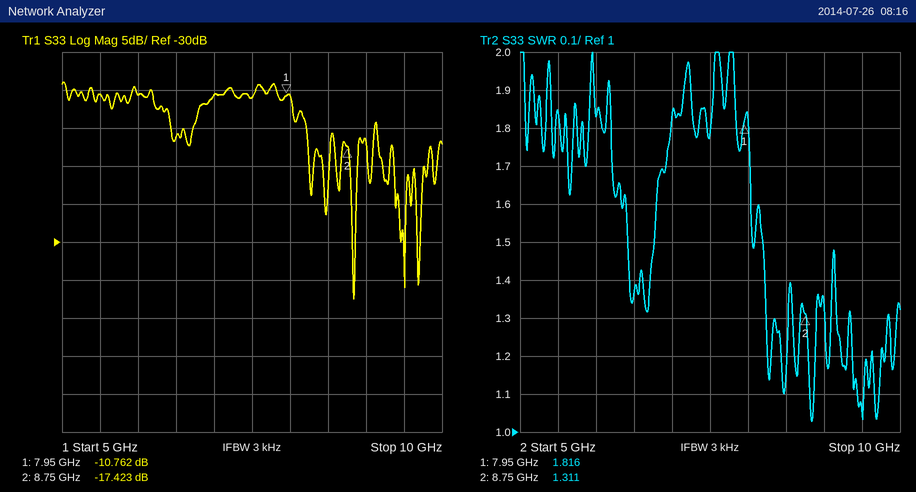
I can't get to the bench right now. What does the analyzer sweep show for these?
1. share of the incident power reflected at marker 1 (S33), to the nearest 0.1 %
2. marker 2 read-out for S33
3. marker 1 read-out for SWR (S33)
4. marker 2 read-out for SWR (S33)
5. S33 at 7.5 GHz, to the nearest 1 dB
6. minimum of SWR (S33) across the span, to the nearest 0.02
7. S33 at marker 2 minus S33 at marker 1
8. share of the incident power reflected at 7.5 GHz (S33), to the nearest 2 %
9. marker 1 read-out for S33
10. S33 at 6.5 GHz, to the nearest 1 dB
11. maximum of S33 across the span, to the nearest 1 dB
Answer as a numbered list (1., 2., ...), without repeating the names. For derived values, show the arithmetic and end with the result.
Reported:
1. 10^(-10.762/10) ≈ 8.4 %
2. -17.423 dB
3. 1.816
4. 1.311
5. -11 dB
6. 1.02
7. -17.423 − (-10.762) = -6.661 dB
8. 10^(-11/10) ≈ 8 %
9. -10.762 dB
10. -16 dB
11. -9 dB
